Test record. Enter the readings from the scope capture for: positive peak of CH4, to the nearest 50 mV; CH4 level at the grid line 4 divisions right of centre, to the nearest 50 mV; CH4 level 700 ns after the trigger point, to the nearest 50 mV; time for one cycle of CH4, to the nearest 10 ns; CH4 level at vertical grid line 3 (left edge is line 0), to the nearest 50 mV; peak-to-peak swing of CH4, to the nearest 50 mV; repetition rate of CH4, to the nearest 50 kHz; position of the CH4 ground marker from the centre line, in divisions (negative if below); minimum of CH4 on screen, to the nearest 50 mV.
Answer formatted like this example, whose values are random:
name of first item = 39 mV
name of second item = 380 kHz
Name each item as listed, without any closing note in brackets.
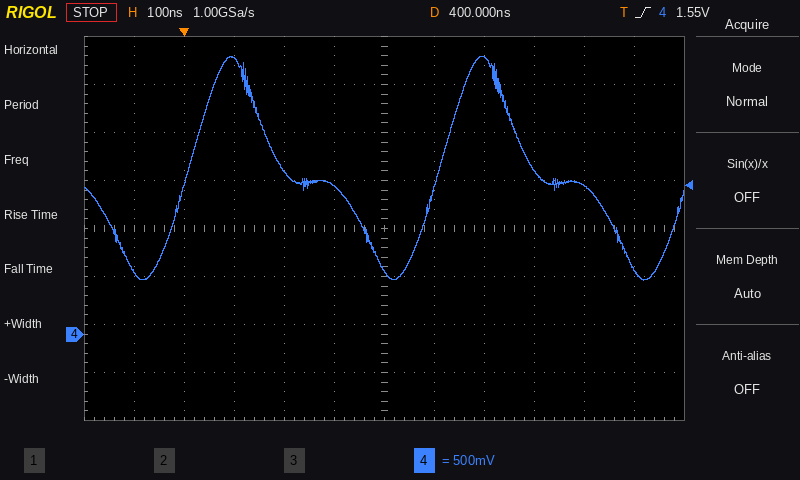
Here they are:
positive peak of CH4, to the nearest 50 mV = 2.90 V
CH4 level at the grid line 4 divisions right of centre, to the nearest 50 mV = 1.55 V
CH4 level 700 ns after the trigger point, to the nearest 50 mV = 1.70 V
time for one cycle of CH4, to the nearest 10 ns = 500 ns
CH4 level at vertical grid line 3 (left edge is line 0), to the nearest 50 mV = 2.85 V
peak-to-peak swing of CH4, to the nearest 50 mV = 2.35 V
repetition rate of CH4, to the nearest 50 kHz = 2.00 MHz
position of the CH4 ground marker from the centre line, in divisions = -2.2 div
minimum of CH4 on screen, to the nearest 50 mV = 550 mV
